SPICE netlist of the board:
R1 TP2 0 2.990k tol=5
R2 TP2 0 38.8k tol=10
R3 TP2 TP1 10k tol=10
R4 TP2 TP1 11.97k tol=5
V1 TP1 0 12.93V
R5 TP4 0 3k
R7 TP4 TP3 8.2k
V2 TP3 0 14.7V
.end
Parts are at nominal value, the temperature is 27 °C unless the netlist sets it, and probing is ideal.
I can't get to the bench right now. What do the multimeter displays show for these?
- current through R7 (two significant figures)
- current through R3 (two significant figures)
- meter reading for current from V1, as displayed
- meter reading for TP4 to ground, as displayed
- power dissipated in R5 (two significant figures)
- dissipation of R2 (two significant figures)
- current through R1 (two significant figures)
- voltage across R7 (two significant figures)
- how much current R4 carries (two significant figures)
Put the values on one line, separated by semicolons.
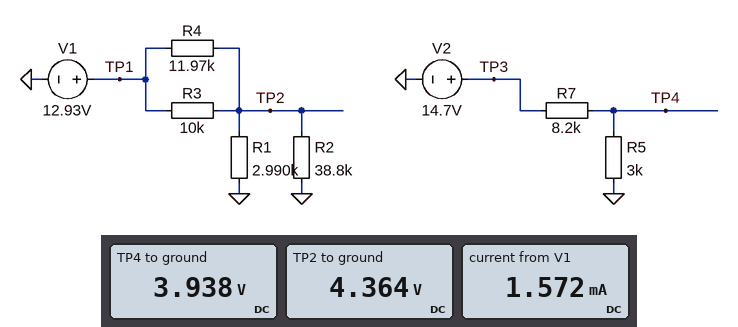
1.3 mA; 860 µA; 1.572 mA; 3.938 V; 5.2 mW; 490 µW; 1.5 mA; 11 V; 720 µA
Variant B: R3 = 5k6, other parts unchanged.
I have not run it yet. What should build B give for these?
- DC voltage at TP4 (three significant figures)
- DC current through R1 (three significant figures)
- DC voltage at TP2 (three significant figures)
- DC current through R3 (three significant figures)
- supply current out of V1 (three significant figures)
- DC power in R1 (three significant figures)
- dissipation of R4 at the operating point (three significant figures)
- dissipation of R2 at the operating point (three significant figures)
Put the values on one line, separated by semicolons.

3.94 V; 1.82 mA; 5.45 V; 1.34 mA; 1.96 mA; 9.92 mW; 4.68 mW; 764 µW
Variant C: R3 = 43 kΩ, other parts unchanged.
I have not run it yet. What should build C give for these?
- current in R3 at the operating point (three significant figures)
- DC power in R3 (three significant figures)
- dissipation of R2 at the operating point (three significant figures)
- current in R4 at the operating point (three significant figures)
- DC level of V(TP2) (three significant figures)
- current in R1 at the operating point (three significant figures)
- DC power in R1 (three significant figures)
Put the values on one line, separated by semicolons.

232 µA; 2.31 mW; 225 µW; 833 µA; 2.96 V; 989 µA; 2.92 mW
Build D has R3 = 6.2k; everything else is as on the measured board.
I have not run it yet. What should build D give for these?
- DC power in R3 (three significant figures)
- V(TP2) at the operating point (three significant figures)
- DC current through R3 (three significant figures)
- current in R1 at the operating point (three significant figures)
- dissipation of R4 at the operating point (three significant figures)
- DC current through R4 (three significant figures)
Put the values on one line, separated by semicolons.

9.56 mW; 5.23 V; 1.24 mA; 1.75 mA; 4.95 mW; 643 µA
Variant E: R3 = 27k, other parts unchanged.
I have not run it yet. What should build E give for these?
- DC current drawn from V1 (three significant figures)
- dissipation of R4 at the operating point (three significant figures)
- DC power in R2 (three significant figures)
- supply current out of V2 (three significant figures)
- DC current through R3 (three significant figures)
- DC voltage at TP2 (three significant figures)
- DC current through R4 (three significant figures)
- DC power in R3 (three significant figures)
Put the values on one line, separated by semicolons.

1.17 mA; 7.84 mW; 271 µW; 1.31 mA; 359 µA; 3.24 V; 809 µA; 3.48 mW
